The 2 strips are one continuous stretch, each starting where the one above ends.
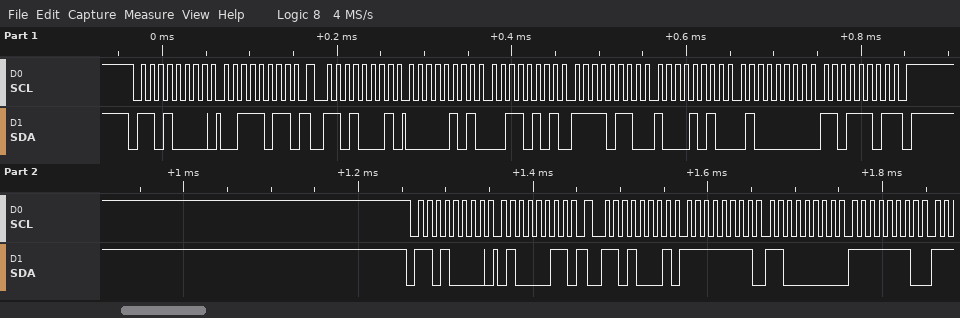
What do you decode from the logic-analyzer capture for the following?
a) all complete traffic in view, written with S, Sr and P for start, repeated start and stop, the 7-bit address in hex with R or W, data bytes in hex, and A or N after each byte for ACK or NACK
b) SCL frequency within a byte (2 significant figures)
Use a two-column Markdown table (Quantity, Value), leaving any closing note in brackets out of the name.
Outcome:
| Quantity | Value |
|---|---|
| all complete traffic in view, written with S, Sr and P for start, repeated start and stop, the 7-bit address in hex with R or W, data bytes in hex, and A or N after each byte for ACK or NACK | S 68W A 3B A Sr 68R A 05 A 35 A F6 A 8A A 40 A DD N P S 68W A 43 A Sr 68R A FF A C0 A FE A |
| SCL frequency within a byte | 100 kHz |
